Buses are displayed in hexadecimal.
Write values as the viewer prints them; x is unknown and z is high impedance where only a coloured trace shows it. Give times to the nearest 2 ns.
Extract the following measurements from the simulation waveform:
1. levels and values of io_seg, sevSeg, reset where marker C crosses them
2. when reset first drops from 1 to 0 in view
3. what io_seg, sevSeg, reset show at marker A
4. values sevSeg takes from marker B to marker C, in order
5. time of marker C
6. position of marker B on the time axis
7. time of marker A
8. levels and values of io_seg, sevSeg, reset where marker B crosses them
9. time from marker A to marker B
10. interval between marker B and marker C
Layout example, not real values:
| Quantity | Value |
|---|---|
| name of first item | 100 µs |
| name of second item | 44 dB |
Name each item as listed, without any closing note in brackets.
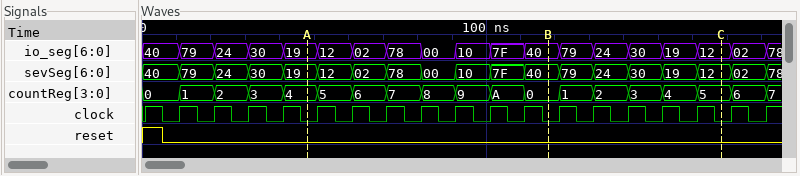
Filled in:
| Quantity | Value |
|---|---|
| levels and values of io_seg, sevSeg, reset where marker C crosses them | io_seg=12, sevSeg=12, reset=0 |
| when reset first drops from 1 to 0 in view | 6 ns |
| what io_seg, sevSeg, reset show at marker A | io_seg=19, sevSeg=19, reset=0 |
| values sevSeg takes from marker B to marker C, in order | 40, 79, 24, 30, 19, 12 |
| time of marker C | 168 ns |
| position of marker B on the time axis | 118 ns |
| time of marker A | 48 ns |
| levels and values of io_seg, sevSeg, reset where marker B crosses them | io_seg=40, sevSeg=40, reset=0 |
| time from marker A to marker B | 70 ns |
| interval between marker B and marker C | 50 ns |
